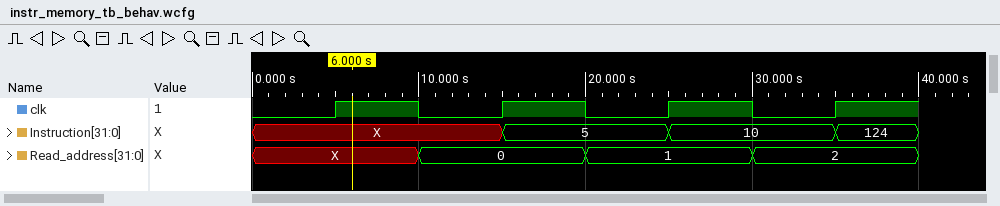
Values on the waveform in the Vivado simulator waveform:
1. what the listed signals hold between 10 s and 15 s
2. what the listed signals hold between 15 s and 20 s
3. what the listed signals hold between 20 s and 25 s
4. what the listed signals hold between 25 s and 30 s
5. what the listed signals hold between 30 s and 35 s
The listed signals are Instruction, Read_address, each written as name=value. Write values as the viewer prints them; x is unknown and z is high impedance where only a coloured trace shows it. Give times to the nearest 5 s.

Instruction=X, Read_address=0
Instruction=5, Read_address=0
Instruction=5, Read_address=1
Instruction=10, Read_address=1
Instruction=10, Read_address=2
